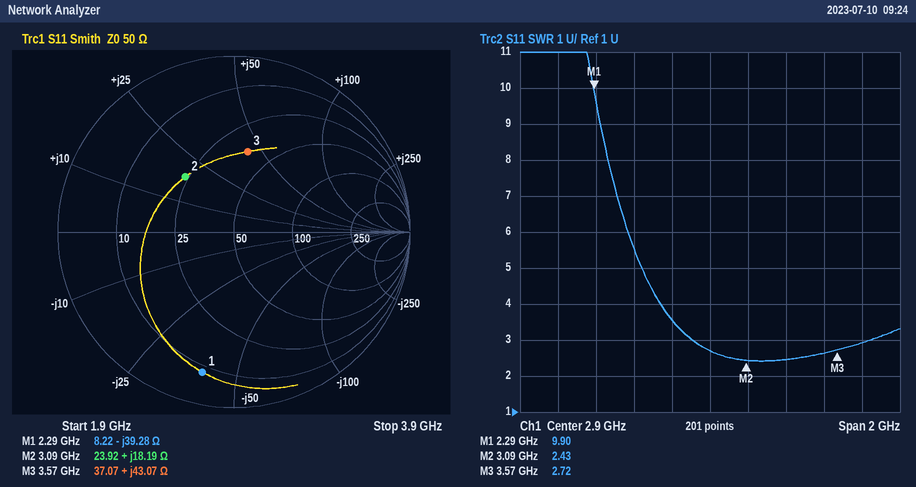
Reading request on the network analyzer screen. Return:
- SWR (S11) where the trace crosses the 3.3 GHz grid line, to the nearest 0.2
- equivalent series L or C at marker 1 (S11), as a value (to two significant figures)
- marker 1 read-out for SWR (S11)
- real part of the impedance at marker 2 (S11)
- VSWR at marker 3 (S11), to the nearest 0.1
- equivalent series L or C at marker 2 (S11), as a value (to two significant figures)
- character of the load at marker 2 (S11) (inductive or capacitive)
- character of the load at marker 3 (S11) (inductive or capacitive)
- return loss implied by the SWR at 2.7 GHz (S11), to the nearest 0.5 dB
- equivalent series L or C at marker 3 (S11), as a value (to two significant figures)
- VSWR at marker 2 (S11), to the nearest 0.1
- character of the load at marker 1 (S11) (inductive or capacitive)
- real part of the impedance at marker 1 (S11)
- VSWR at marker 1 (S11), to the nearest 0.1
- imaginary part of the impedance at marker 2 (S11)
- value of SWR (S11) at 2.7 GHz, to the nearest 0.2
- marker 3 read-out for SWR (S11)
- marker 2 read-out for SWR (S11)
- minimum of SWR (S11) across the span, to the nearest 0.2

2.4
1.8 pF
9.90
23.92 Ω
2.7
940 pH
inductive
inductive
5.0 dB
1.9 nH
2.4
capacitive
8.22 Ω
9.9
+18.19 Ω
3.6
2.72
2.43
2.4
